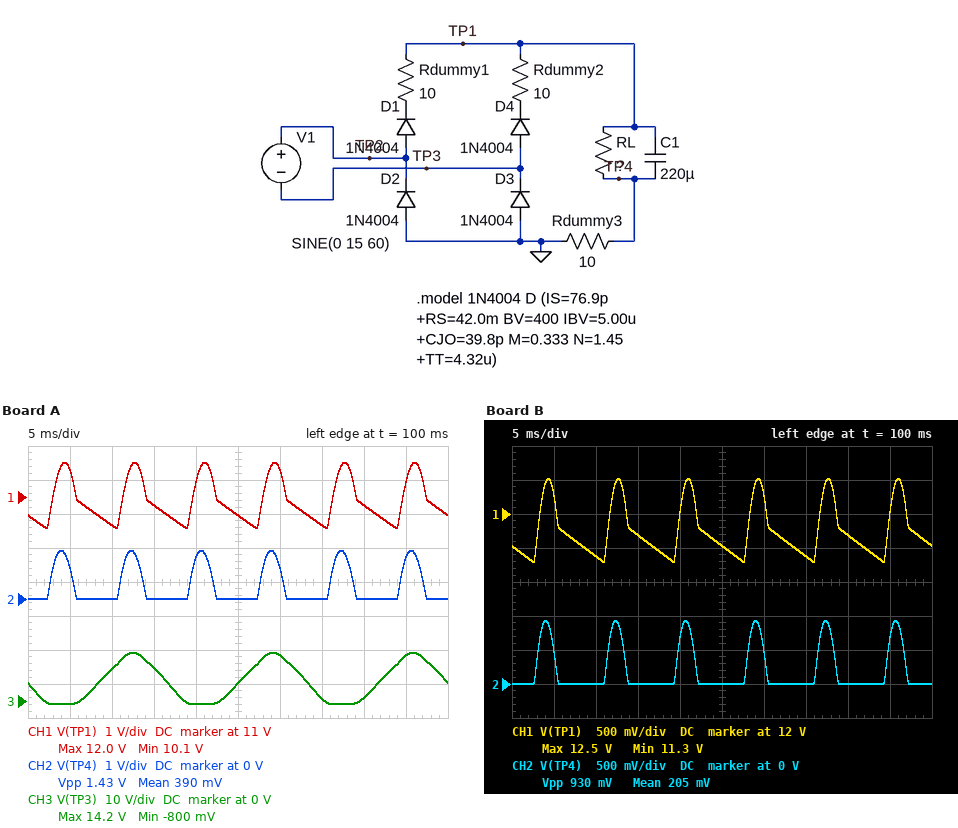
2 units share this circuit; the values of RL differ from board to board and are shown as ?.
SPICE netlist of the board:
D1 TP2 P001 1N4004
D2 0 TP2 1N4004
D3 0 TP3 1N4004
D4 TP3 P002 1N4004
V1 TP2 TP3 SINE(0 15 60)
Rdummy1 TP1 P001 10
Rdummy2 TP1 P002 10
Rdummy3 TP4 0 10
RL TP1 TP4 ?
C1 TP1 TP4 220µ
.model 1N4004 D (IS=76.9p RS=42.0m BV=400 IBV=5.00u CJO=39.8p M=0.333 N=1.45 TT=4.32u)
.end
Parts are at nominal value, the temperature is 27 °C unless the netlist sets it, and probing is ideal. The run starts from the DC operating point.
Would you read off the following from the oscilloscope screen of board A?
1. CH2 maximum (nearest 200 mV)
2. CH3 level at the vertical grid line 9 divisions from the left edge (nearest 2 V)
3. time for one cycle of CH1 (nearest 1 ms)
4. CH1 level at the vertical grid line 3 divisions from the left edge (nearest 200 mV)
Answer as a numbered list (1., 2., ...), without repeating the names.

1. 1.4 V
2. 14 V
3. 8 ms
4. 10.8 V
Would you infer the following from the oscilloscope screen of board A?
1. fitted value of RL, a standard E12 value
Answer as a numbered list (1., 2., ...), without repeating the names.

1. 270 Ω
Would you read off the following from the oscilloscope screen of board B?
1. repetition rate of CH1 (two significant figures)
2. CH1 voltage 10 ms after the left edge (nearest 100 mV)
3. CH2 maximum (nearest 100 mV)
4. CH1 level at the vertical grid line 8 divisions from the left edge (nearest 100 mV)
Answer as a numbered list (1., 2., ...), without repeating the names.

1. 120 Hz
2. 11.4 V
3. 900 mV
4. 11.7 V
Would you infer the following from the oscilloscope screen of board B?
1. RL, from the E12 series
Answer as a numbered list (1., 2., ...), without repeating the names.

1. 560 Ω
